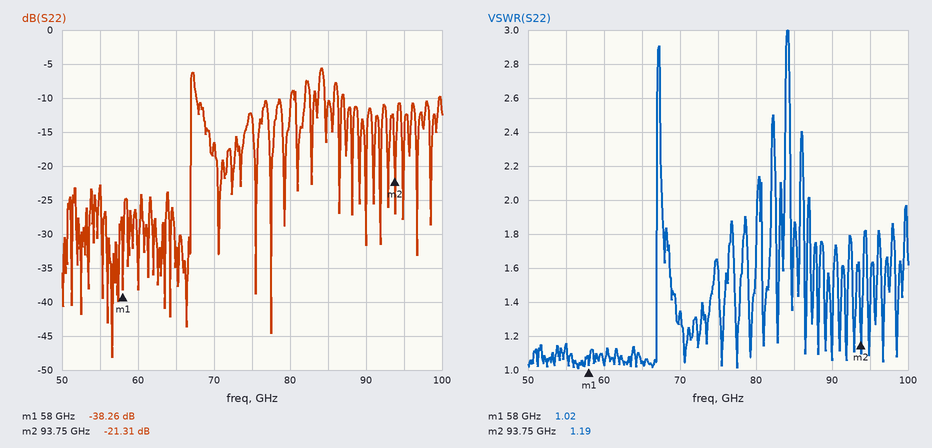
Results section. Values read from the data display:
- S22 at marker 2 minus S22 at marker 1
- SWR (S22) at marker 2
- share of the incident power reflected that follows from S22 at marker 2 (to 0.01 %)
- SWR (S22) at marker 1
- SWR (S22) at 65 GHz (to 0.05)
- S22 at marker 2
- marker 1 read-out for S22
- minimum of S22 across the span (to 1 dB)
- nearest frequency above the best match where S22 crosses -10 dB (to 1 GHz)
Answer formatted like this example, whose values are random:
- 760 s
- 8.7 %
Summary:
- 16.95 dB
- 1.19
- 0.74 %
- 1.02
- 1.05
- -21.31 dB
- -38.26 dB
- -48 dB
- 67 GHz
